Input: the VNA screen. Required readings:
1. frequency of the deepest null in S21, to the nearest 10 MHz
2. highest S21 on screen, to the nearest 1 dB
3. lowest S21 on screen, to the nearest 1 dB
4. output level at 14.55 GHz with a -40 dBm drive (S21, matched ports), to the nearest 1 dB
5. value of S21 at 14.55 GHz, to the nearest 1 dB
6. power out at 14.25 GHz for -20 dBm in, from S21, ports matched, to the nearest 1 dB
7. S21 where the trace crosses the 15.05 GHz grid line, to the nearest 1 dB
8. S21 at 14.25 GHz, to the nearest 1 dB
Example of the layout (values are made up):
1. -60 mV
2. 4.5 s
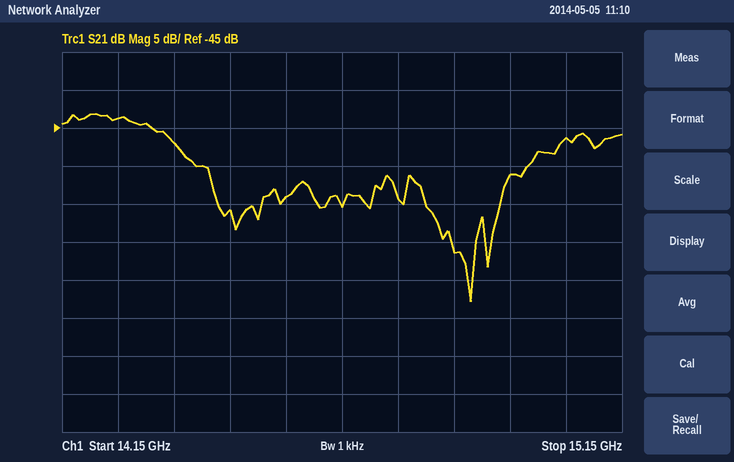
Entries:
1. 14.88 GHz
2. -43 dB
3. -68 dB
4. -94 dBm
5. -54 dB
6. -64 dBm
7. -46 dB
8. -44 dB
